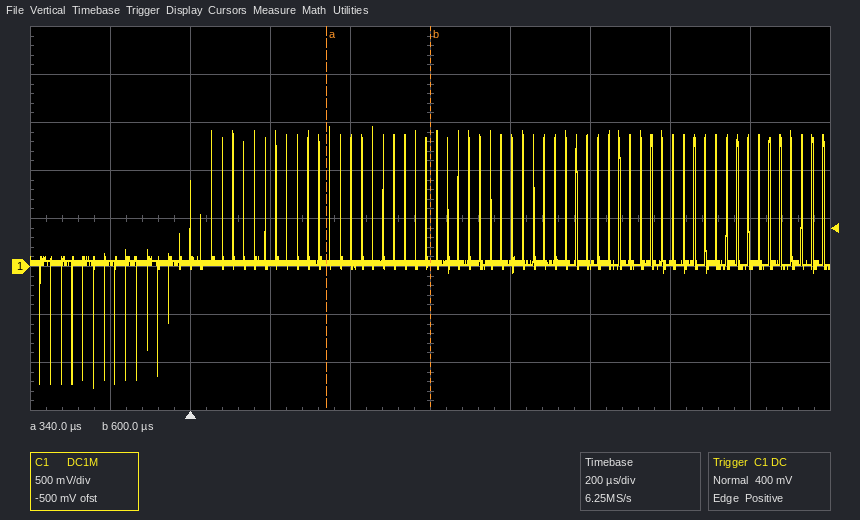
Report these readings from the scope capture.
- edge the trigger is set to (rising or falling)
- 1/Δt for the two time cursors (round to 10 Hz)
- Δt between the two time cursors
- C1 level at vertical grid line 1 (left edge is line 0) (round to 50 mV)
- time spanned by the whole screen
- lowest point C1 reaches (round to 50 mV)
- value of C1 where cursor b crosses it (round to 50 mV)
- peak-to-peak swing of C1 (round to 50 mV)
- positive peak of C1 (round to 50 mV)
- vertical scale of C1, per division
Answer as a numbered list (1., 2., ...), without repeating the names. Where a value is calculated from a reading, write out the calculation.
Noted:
1. rising
2. 1 / 260 µs ≈ 3.85 kHz
3. 600 µs − (340 µs) = 260 µs
4. 50 mV
5. 2 ms
6. -1.25 V
7. 50 mV
8. 1.45 V − (-1.25 V) = 2.70 V
9. 1.45 V
10. 500 mV
